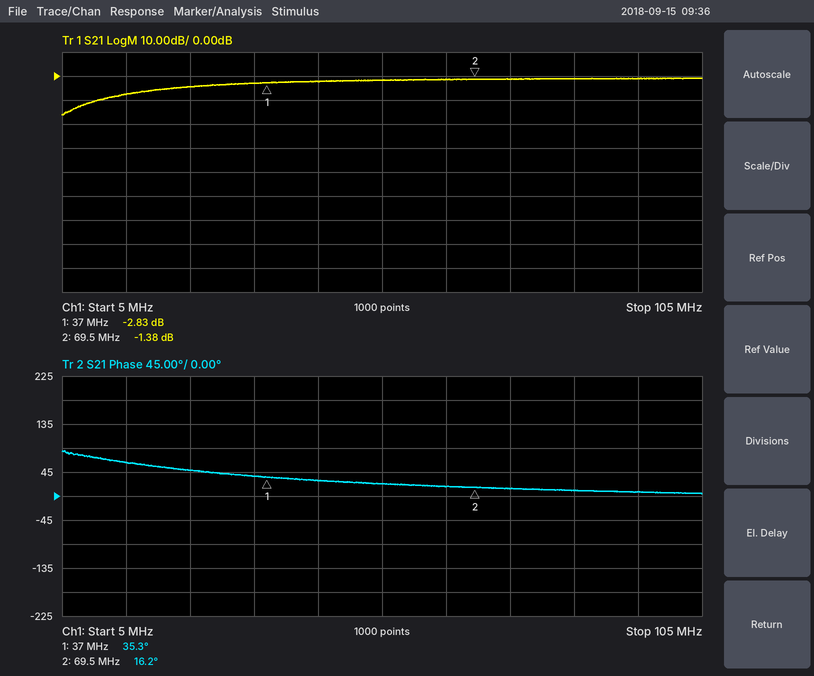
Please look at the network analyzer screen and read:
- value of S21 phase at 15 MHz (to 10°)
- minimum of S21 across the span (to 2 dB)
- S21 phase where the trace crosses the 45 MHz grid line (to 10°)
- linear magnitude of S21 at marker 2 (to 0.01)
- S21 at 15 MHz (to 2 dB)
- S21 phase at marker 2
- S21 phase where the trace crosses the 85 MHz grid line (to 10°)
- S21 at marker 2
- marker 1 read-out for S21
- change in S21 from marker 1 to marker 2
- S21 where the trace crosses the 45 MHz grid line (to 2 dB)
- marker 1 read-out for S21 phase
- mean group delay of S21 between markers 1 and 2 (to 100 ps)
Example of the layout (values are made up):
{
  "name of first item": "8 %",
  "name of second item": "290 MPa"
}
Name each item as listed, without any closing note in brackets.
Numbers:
{
  "value of S21 phase at 15 MHz": "60°",
  "minimum of S21 across the span": "-16 dB",
  "S21 phase where the trace crosses the 45 MHz grid line": "30°",
  "linear magnitude of S21 at marker 2": "0.85",
  "S21 at 15 MHz": "-8 dB",
  "S21 phase at marker 2": "16.2°",
  "S21 phase where the trace crosses the 85 MHz grid line": "10°",
  "S21 at marker 2": "-1.38 dB",
  "marker 1 read-out for S21": "-2.83 dB",
  "change in S21 from marker 1 to marker 2": "1.45 dB",
  "S21 where the trace crosses the 45 MHz grid line": "-2 dB",
  "marker 1 read-out for S21 phase": "35.3°",
  "mean group delay of S21 between markers 1 and 2": "1.6 ns"
}
